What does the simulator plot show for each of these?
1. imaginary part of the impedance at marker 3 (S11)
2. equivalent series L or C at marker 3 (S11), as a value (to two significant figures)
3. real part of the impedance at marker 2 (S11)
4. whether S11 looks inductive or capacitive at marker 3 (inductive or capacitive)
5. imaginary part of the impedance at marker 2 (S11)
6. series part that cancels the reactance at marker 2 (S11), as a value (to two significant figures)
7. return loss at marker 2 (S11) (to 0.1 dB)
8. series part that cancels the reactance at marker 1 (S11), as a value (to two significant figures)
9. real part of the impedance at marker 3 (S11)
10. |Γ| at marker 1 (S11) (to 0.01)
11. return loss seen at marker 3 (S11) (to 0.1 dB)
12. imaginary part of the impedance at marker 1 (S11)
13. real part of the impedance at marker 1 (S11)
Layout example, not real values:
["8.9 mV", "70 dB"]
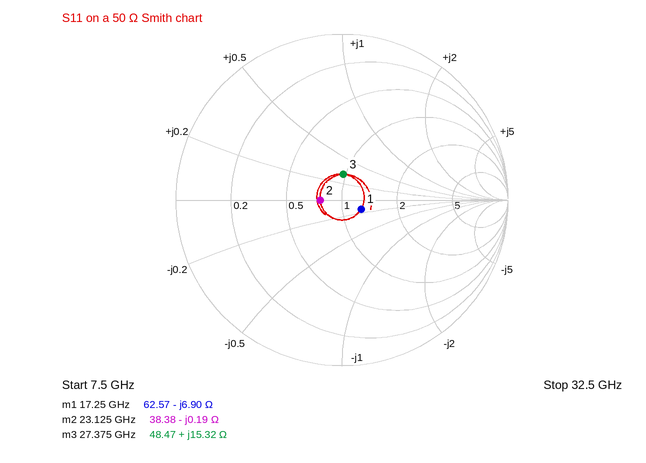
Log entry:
["+15.32 Ω", "89 pH", "38.38 Ω", "inductive", "-0.19 Ω", "1.3 pH", "17.6 dB", "64 pH", "48.47 Ω", "0.13", "16.2 dB", "-6.90 Ω", "62.57 Ω"]
